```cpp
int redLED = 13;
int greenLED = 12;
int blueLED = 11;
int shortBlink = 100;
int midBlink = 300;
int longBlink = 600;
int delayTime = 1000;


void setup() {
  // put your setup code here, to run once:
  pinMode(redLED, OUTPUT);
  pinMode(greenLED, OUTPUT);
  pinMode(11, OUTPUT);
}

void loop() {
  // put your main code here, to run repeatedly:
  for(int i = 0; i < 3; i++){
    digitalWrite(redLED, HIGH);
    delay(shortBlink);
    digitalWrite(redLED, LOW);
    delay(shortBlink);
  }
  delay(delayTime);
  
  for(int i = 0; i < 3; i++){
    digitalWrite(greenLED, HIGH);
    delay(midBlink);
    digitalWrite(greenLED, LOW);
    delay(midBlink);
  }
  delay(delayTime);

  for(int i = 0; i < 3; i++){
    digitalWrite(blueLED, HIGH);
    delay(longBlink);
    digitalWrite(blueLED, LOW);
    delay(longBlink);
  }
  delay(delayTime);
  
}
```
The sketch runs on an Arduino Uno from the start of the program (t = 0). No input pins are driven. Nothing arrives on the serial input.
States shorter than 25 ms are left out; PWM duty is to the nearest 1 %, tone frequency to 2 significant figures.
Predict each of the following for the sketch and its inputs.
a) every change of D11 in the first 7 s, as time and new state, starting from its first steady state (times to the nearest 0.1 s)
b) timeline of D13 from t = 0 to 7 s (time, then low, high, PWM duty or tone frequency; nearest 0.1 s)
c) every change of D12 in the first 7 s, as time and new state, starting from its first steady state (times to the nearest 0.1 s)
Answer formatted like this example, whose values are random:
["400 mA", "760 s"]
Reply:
["0 s low; 4.4 s high; 5 s low; 5.6 s high; 6.2 s low; 6.8 s high", "0 s high; 0.1 s low; 0.2 s high; 0.3 s low; 0.4 s high; 0.5 s low", "0 s low; 1.6 s high; 1.9 s low; 2.2 s high; 2.5 s low; 2.8 s high; 3.1 s low"]
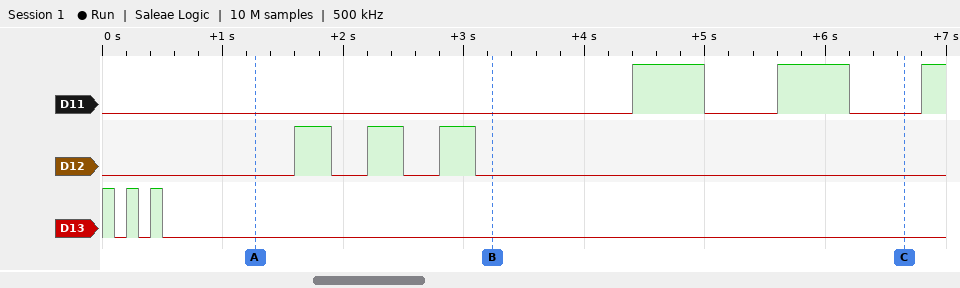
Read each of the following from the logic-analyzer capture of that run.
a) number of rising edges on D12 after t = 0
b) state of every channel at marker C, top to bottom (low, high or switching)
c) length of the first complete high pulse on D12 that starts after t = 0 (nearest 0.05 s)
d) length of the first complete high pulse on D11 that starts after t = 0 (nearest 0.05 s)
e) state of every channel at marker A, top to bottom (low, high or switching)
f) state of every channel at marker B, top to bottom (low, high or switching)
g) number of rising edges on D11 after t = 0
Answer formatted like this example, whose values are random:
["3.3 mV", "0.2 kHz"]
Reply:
["3", "D11 low, D12 low, D13 low", "0.30 s", "0.60 s", "D11 low, D12 low, D13 low", "D11 low, D12 low, D13 low", "3"]
